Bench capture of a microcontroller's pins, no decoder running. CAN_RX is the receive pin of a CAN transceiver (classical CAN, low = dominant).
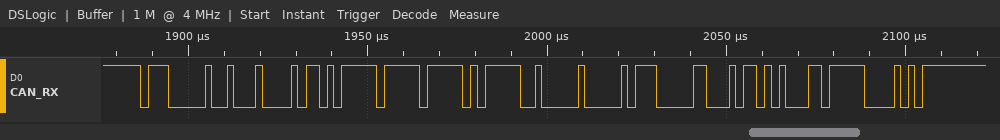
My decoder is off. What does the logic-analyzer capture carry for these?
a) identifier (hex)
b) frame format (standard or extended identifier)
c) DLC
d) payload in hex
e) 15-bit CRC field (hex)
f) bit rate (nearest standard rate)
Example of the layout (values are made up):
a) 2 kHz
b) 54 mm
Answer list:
a) 0x701
b) standard
c) 8
d) 5A FF FF 7D 00 1C 11 6A
e) 0x1BE2
f) 500 kbit/s
